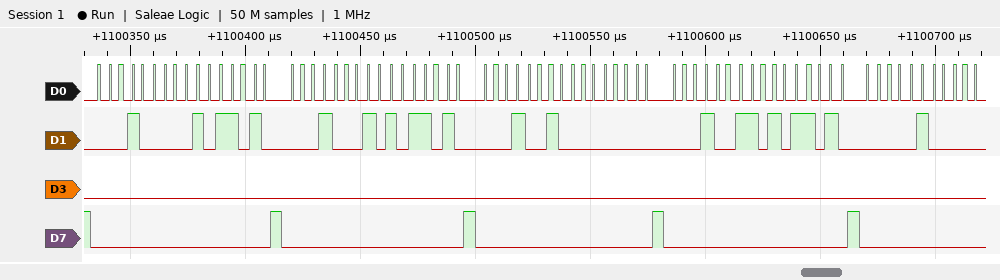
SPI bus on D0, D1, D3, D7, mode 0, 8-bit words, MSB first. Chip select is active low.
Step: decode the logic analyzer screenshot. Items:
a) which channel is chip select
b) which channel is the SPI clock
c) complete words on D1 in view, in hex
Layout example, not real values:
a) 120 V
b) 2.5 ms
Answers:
a) D7
b) D0
c) 10, 5A, 11, 5A, 12, 00, 13, 5A, 04
